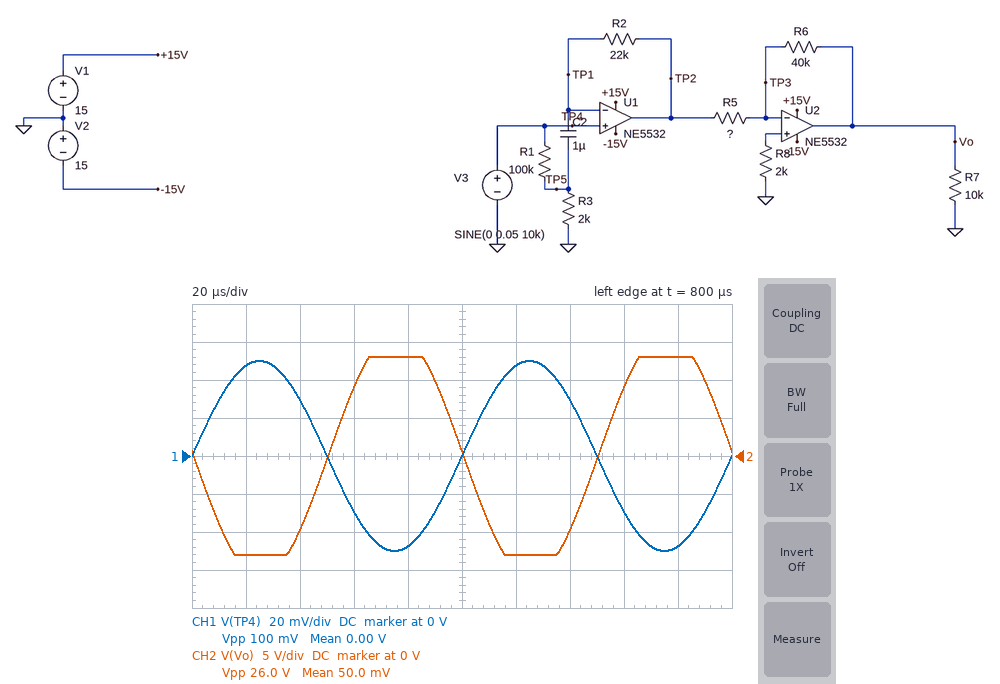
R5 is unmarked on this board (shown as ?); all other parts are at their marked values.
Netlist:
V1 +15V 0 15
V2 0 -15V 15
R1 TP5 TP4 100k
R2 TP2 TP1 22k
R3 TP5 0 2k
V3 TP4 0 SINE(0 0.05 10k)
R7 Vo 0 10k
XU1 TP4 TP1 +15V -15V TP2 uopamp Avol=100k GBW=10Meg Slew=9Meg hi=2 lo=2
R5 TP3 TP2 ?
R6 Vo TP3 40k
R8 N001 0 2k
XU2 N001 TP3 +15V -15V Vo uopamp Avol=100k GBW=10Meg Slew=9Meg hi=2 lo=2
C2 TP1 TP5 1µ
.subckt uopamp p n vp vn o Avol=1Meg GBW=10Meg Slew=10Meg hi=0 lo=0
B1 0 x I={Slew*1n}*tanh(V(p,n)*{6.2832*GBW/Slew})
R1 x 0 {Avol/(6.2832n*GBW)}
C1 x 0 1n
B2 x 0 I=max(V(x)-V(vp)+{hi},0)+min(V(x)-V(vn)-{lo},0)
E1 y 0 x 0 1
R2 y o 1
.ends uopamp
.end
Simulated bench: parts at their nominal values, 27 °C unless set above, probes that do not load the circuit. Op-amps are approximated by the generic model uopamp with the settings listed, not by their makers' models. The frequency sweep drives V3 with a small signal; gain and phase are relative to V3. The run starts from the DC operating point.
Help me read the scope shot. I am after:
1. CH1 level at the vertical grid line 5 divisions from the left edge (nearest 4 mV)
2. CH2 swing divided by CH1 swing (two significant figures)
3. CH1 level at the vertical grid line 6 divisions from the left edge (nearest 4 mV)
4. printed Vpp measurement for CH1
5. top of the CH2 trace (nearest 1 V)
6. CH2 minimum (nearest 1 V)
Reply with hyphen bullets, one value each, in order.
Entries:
- 0 V
- 260
- 48 mV
- 100 mV
- 13 V
- -13 V
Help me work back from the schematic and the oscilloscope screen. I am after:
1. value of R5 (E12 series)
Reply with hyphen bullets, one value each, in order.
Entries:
- 1.5 kΩ
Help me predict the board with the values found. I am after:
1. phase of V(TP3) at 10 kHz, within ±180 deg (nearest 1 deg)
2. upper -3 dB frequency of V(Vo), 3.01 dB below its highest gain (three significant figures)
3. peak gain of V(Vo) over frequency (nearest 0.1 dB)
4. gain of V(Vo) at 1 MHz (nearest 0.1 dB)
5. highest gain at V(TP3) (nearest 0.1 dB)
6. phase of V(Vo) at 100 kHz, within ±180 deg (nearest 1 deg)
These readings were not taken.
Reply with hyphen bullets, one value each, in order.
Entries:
- 88 deg
- 312 kHz
- 50.1 dB
- 36.8 dB
- 18.1 dB
- 158 deg
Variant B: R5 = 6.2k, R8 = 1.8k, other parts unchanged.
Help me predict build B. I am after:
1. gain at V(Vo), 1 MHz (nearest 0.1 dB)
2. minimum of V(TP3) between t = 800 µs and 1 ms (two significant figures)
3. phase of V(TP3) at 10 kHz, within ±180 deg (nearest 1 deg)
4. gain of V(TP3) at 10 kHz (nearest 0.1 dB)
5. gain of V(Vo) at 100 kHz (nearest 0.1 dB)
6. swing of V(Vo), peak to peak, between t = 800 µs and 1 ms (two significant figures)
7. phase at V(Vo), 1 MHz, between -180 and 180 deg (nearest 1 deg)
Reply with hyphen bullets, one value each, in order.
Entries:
- 31.9 dB
- -3.9 mV
- 89 deg
- -22.2 dB
- 37.7 dB
- 7.7 V
- 93 deg
